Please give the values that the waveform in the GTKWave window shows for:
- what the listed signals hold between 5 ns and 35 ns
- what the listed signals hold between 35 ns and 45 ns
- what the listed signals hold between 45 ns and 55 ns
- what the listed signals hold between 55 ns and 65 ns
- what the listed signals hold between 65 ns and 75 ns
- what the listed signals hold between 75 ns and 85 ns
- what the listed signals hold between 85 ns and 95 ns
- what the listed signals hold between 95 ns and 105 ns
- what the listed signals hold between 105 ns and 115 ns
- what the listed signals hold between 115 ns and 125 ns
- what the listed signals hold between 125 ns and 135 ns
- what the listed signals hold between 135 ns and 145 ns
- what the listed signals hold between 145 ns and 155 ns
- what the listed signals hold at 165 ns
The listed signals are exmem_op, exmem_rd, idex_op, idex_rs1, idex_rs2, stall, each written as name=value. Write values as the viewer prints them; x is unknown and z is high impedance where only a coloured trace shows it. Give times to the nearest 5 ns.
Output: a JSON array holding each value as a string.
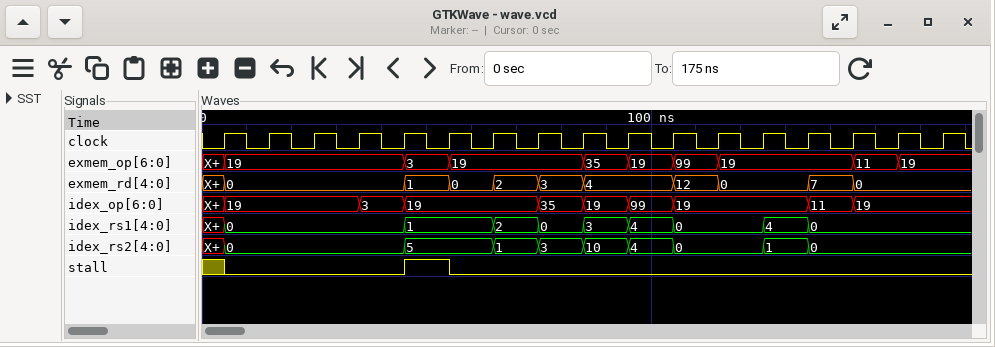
["exmem_op=19, exmem_rd=0, idex_op=19, idex_rs1=0, idex_rs2=0, stall=0", "exmem_op=19, exmem_rd=0, idex_op=3, idex_rs1=0, idex_rs2=0, stall=0", "exmem_op=3, exmem_rd=1, idex_op=19, idex_rs1=1, idex_rs2=5, stall=1", "exmem_op=19, exmem_rd=0, idex_op=19, idex_rs1=1, idex_rs2=5, stall=0", "exmem_op=19, exmem_rd=2, idex_op=19, idex_rs1=2, idex_rs2=1, stall=0", "exmem_op=19, exmem_rd=3, idex_op=35, idex_rs1=0, idex_rs2=3, stall=0", "exmem_op=35, exmem_rd=4, idex_op=19, idex_rs1=3, idex_rs2=10, stall=0", "exmem_op=19, exmem_rd=4, idex_op=99, idex_rs1=4, idex_rs2=4, stall=0", "exmem_op=99, exmem_rd=12, idex_op=19, idex_rs1=0, idex_rs2=0, stall=0", "exmem_op=19, exmem_rd=0, idex_op=19, idex_rs1=0, idex_rs2=0, stall=0", "exmem_op=19, exmem_rd=0, idex_op=19, idex_rs1=4, idex_rs2=1, stall=0", "exmem_op=19, exmem_rd=7, idex_op=11, idex_rs1=0, idex_rs2=0, stall=0", "exmem_op=11, exmem_rd=0, idex_op=19, idex_rs1=0, idex_rs2=0, stall=0", "exmem_op=19, exmem_rd=0, idex_op=19, idex_rs1=0, idex_rs2=0, stall=0"]
